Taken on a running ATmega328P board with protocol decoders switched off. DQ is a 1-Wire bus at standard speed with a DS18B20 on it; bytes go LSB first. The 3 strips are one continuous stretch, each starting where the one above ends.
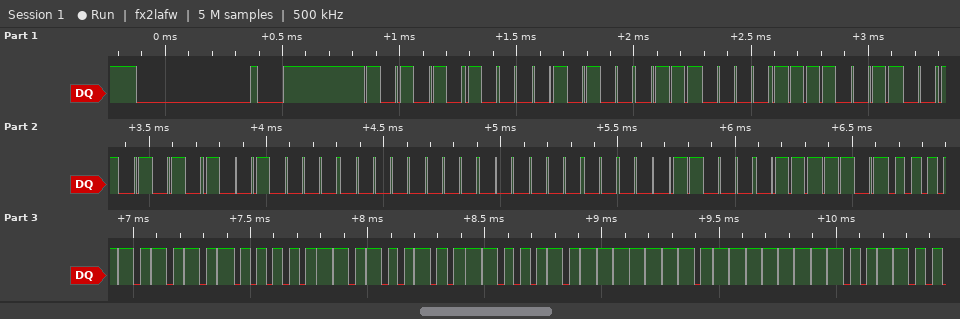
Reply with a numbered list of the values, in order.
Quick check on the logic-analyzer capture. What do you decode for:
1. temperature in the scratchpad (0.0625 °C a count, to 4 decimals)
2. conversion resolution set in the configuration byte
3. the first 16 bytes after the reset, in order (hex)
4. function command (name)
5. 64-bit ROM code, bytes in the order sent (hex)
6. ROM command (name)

1. 85.0000 °C
2. 12 bits
3. 55 28 0E CF 54 09 00 00 18 BE 50 05 4B 46 7F FF
4. Read Scratchpad
5. 28 0E CF 54 09 00 00 18
6. Match ROM
